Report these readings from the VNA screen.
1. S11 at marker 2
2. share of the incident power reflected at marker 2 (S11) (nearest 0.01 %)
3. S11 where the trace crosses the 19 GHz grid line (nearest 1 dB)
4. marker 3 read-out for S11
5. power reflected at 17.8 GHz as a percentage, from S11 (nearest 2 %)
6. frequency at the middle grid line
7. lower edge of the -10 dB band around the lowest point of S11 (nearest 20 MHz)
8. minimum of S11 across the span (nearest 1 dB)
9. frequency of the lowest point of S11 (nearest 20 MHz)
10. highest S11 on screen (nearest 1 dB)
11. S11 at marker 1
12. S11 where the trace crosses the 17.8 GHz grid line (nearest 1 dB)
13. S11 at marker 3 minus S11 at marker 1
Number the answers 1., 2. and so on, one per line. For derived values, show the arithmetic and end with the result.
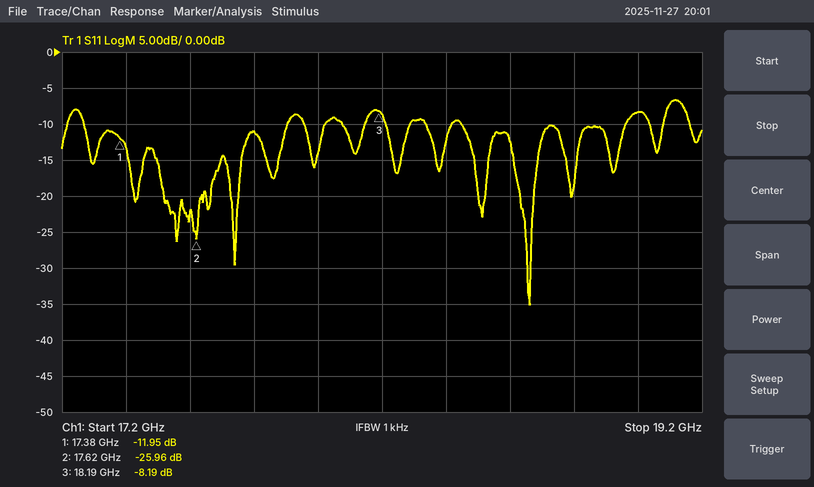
1. -25.96 dB
2. 10^(-25.96/10) ≈ 0.25 %
3. -8 dB
4. -8.19 dB
5. 10^(-11/10) ≈ 8 %
6. 18.2 GHz
7. 18.44 GHz
8. -35 dB
9. 18.66 GHz
10. -7 dB
11. -11.95 dB
12. -11 dB
13. -8.19 − (-11.95) = 3.76 dB
